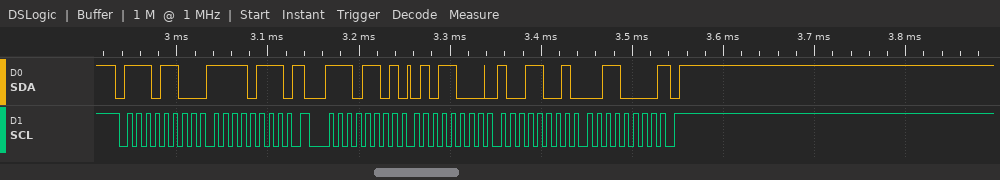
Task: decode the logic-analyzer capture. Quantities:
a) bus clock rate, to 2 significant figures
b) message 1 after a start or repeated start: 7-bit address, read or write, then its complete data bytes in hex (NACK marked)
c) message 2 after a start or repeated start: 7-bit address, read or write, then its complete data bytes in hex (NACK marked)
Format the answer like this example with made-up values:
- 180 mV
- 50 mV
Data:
- 100 kHz
- 0x76 write: F7
- 0x76 read: 58 99 30 NACK
